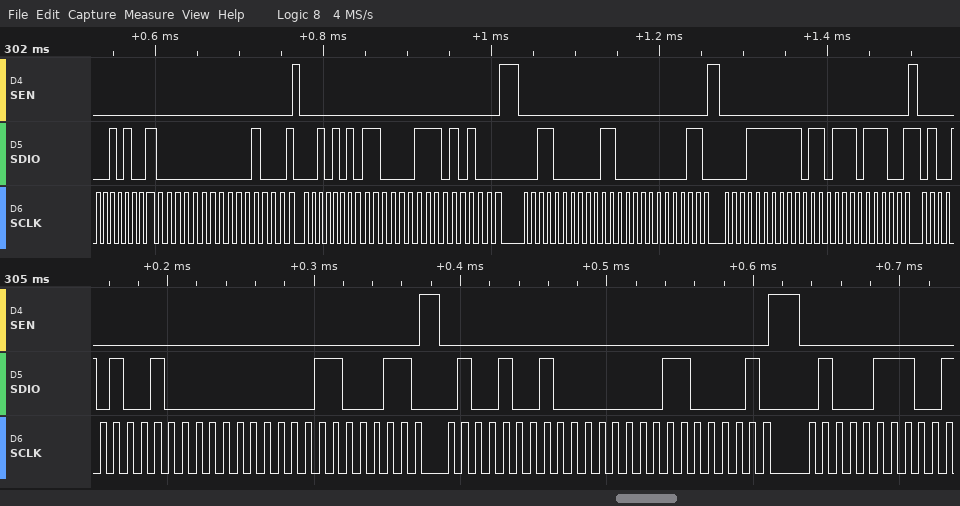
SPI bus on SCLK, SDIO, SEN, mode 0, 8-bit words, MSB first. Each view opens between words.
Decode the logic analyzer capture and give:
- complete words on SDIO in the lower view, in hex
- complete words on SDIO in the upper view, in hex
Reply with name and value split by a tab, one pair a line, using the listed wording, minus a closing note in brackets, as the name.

complete words on SDIO in the lower view, in hex	48, 00, C6, 49, 00, C2, 47
complete words on SDIO in the upper view, in hex	29, 00, 11, 2A, C3, A8, 30, 30, 06, 1F, DB, B9
